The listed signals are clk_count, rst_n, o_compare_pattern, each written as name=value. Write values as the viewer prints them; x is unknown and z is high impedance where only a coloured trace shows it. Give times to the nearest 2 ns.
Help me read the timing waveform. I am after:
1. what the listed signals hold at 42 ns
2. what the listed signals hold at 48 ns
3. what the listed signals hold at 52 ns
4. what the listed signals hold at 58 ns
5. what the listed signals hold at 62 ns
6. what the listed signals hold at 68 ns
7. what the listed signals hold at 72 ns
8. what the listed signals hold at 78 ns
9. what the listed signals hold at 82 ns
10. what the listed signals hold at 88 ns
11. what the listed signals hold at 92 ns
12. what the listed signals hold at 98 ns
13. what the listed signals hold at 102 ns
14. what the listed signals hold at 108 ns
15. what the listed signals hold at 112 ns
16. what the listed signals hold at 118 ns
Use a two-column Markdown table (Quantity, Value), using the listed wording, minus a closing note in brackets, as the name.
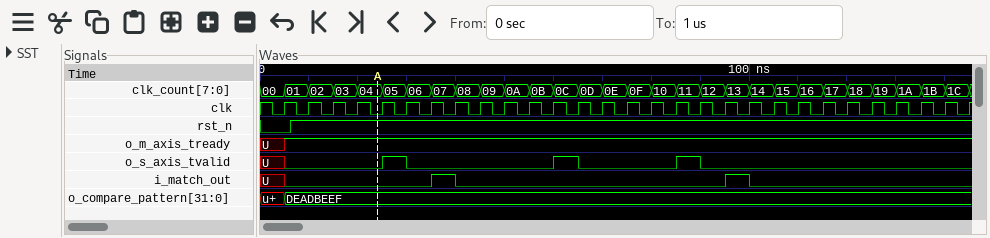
| Quantity | Value |
|---|---|
| what the listed signals hold at 42 ns | clk_count=08, rst_n=1, o_compare_pattern=DEADBEEF |
| what the listed signals hold at 48 ns | clk_count=09, rst_n=1, o_compare_pattern=DEADBEEF |
| what the listed signals hold at 52 ns | clk_count=0A, rst_n=1, o_compare_pattern=DEADBEEF |
| what the listed signals hold at 58 ns | clk_count=0B, rst_n=1, o_compare_pattern=DEADBEEF |
| what the listed signals hold at 62 ns | clk_count=0C, rst_n=1, o_compare_pattern=DEADBEEF |
| what the listed signals hold at 68 ns | clk_count=0D, rst_n=1, o_compare_pattern=DEADBEEF |
| what the listed signals hold at 72 ns | clk_count=0E, rst_n=1, o_compare_pattern=DEADBEEF |
| what the listed signals hold at 78 ns | clk_count=0F, rst_n=1, o_compare_pattern=DEADBEEF |
| what the listed signals hold at 82 ns | clk_count=10, rst_n=1, o_compare_pattern=DEADBEEF |
| what the listed signals hold at 88 ns | clk_count=11, rst_n=1, o_compare_pattern=DEADBEEF |
| what the listed signals hold at 92 ns | clk_count=12, rst_n=1, o_compare_pattern=DEADBEEF |
| what the listed signals hold at 98 ns | clk_count=13, rst_n=1, o_compare_pattern=DEADBEEF |
| what the listed signals hold at 102 ns | clk_count=14, rst_n=1, o_compare_pattern=DEADBEEF |
| what the listed signals hold at 108 ns | clk_count=15, rst_n=1, o_compare_pattern=DEADBEEF |
| what the listed signals hold at 112 ns | clk_count=16, rst_n=1, o_compare_pattern=DEADBEEF |
| what the listed signals hold at 118 ns | clk_count=17, rst_n=1, o_compare_pattern=DEADBEEF |
